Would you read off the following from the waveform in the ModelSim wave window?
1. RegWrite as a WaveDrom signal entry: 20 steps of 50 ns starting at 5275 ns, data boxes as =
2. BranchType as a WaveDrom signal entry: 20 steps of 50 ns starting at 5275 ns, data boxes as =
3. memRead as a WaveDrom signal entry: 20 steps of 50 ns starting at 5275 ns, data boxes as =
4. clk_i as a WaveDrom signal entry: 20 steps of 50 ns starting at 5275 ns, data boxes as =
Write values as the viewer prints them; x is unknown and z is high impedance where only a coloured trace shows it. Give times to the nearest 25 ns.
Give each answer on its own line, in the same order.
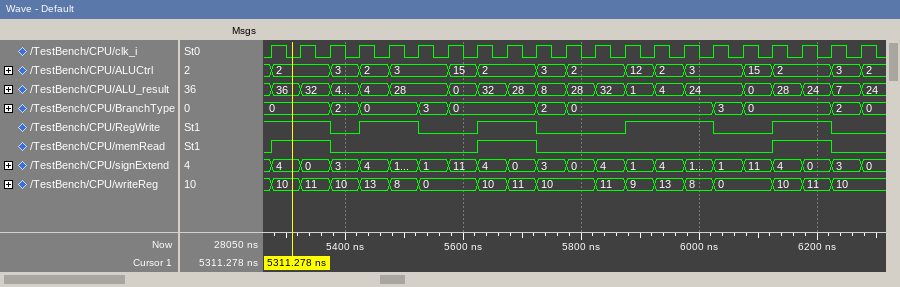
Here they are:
{name: 'RegWrite', wave: '1.01.0.1.0..1..0.1.0'}
{name: 'BranchType', wave: '=.==.==..==....==..=', data: '0 2 0 3 0 2 0 3 0 2'}
{name: 'memRead', wave: '1.0....1.0.......1.0'}
{name: 'clk_i', wave: 'p...................'}
